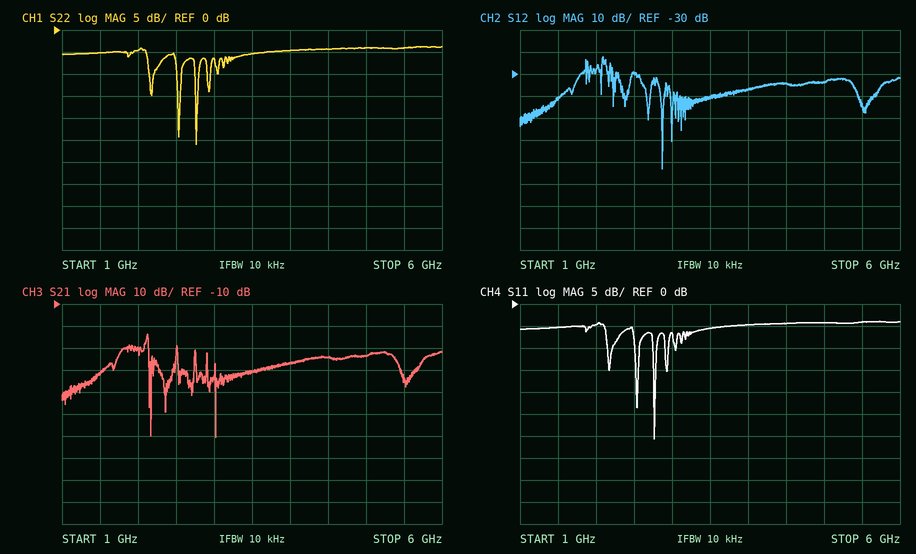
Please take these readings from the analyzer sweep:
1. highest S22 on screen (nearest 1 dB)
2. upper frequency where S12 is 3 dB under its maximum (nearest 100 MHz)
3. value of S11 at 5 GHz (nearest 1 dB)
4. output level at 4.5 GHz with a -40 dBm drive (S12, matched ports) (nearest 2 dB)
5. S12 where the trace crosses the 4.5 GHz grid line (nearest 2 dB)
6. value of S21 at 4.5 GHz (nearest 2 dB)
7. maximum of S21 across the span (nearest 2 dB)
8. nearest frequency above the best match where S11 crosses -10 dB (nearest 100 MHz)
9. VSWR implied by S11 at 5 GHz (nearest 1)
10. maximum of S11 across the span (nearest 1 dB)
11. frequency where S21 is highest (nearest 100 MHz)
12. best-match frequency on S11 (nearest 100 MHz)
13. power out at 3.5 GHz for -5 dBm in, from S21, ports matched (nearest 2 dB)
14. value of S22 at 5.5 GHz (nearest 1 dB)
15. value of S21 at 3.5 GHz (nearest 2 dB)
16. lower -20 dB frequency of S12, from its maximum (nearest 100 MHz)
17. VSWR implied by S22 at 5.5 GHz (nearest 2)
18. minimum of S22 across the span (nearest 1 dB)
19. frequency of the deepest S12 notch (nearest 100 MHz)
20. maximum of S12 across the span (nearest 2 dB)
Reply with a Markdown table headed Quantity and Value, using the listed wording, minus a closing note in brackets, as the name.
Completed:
| Quantity | Value |
|---|---|
| highest S22 on screen | -4 dB |
| upper frequency where S12 is 3 dB under its maximum | 2.1 GHz |
| value of S11 at 5 GHz | -4 dB |
| output level at 4.5 GHz with a -40 dBm drive (S12, matched ports) | -74 dBm |
| S12 where the trace crosses the 4.5 GHz grid line | -34 dB |
| value of S21 at 4.5 GHz | -34 dB |
| maximum of S21 across the span | -24 dB |
| nearest frequency above the best match where S11 crosses -10 dB | 2.8 GHz |
| VSWR implied by S11 at 5 GHz | 4 |
| maximum of S11 across the span | -4 dB |
| frequency where S21 is highest | 2.1 GHz |
| best-match frequency on S11 | 2.8 GHz |
| power out at 3.5 GHz for -5 dBm in, from S21, ports matched | -46 dBm |
| value of S22 at 5.5 GHz | -4 dB |
| value of S21 at 3.5 GHz | -40 dB |
| lower -20 dB frequency of S12, from its maximum | 1.5 GHz |
| VSWR implied by S22 at 5.5 GHz | 4 |
| minimum of S22 across the span | -26 dB |
| frequency of the deepest S12 notch | 2.9 GHz |
| maximum of S12 across the span | -22 dB |
